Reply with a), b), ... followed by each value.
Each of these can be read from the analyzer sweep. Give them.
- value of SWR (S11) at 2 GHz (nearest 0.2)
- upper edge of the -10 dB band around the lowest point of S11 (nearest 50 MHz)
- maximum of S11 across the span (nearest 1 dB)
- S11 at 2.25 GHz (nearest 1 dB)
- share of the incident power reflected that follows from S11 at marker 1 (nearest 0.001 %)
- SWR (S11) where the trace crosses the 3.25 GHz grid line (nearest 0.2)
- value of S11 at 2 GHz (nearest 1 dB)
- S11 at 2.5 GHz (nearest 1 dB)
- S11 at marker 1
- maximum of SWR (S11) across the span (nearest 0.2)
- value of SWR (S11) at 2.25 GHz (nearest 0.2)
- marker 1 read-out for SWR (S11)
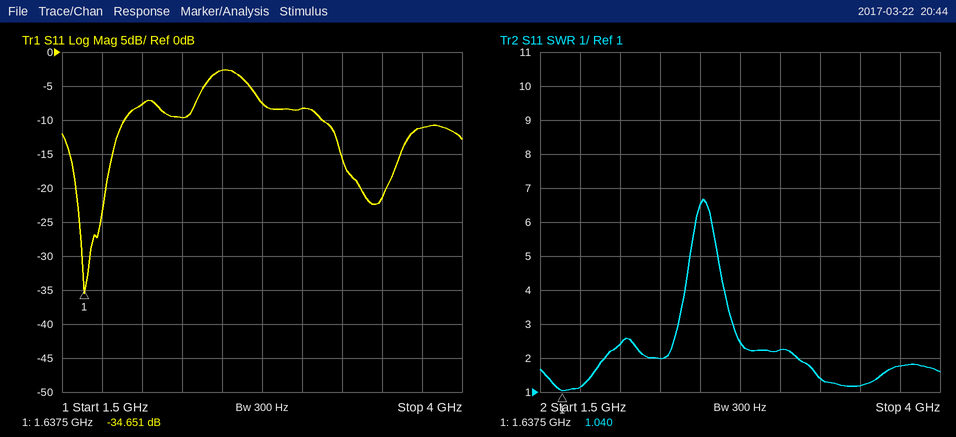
a) 2.4
b) 1.90 GHz
c) -3 dB
d) -10 dB
e) 0.034 %
f) 1.4
g) -8 dB
h) -3 dB
i) -34.651 dB
j) 6.6
k) 2.0
l) 1.040
